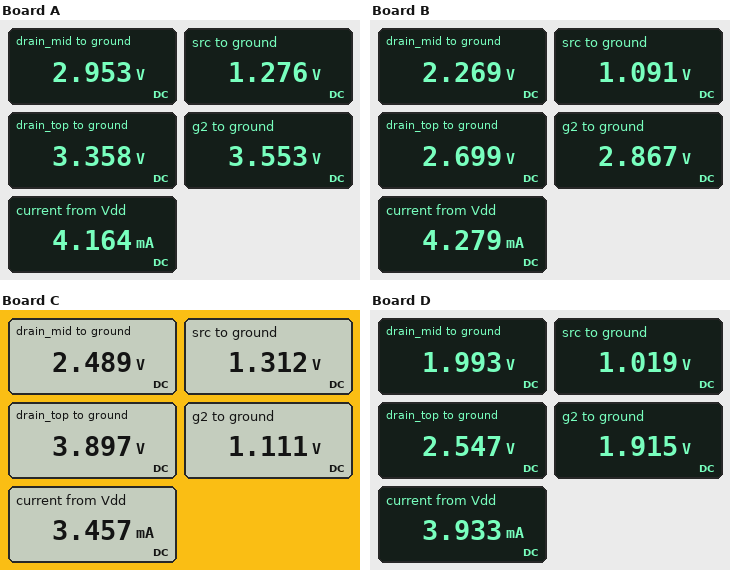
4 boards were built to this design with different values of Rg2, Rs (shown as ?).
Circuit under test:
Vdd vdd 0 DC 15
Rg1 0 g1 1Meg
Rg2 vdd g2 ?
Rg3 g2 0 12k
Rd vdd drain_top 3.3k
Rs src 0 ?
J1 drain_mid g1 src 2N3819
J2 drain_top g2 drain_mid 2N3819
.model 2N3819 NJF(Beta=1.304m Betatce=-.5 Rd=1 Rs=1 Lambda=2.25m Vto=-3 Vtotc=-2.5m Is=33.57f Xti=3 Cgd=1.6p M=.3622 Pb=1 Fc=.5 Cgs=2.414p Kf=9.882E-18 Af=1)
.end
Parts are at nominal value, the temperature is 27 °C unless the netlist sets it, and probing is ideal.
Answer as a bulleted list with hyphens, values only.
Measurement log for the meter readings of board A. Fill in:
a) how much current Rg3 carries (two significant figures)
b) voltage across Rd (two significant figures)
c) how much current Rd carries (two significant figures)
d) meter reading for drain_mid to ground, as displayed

- 300 µA
- 12 V
- 3.5 mA
- 2.953 V
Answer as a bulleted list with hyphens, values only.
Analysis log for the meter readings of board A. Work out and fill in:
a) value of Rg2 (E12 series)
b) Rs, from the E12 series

- 18 kΩ
- 330 Ω
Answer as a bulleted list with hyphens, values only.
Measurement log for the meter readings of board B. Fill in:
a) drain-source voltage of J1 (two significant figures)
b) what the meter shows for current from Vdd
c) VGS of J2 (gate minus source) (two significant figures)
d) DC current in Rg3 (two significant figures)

- 1.2 V
- 4.279 mA
- 600 mV
- 240 µA
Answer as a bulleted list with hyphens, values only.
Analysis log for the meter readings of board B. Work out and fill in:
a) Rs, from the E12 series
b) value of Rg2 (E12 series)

- 270 Ω
- 22 kΩ
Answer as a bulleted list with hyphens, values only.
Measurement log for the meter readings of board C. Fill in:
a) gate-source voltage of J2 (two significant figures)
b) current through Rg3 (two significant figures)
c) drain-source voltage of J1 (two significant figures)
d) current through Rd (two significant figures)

- -1.4 V
- 93 µA
- 1.2 V
- 3.4 mA
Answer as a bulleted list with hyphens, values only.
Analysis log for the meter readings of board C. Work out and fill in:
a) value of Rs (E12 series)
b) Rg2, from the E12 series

- 390 Ω
- 150 kΩ
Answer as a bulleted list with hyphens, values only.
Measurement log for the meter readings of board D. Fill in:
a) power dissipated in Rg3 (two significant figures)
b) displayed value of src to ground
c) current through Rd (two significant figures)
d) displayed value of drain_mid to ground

- 310 µW
- 1.019 V
- 3.8 mA
- 1.993 V
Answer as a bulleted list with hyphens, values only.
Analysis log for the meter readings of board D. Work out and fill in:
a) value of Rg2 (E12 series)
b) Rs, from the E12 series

- 82 kΩ
- 270 Ω
